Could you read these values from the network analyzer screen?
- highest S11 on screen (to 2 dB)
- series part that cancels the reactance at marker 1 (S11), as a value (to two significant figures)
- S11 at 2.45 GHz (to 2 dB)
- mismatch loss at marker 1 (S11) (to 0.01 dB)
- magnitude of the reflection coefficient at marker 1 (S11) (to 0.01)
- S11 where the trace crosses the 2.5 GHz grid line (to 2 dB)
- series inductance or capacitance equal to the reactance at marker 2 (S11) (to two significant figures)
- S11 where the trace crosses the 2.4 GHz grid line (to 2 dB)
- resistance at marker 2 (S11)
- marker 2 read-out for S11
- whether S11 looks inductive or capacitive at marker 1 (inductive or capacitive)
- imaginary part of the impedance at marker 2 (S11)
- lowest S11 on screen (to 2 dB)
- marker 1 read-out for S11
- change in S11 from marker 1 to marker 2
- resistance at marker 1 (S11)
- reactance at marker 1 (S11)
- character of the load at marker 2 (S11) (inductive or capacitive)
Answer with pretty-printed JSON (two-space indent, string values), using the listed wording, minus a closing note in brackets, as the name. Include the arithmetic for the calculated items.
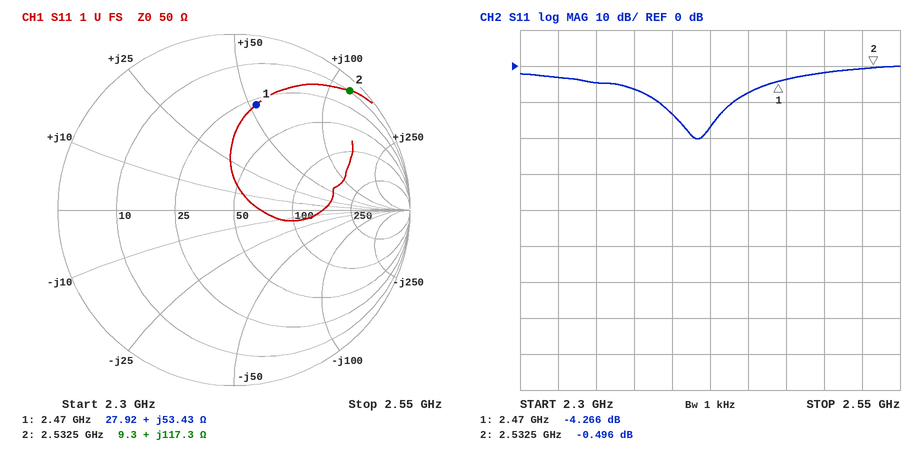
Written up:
{
  "highest S11 on screen": "0 dB",
  "series part that cancels the reactance at marker 1 (S11), as a value": "C = 1/(2π × 2.47 GHz × 53.43 Ω) ≈ 1.2 pF",
  "S11 at 2.45 GHz": "-8 dB",
  "mismatch loss at marker 1 (S11)": "−10 log10(1 − 10^(-4.266/10)) ≈ 2.04 dB",
  "magnitude of the reflection coefficient at marker 1 (S11)": "0.61",
  "S11 where the trace crosses the 2.5 GHz grid line": "-2 dB",
  "series inductance or capacitance equal to the reactance at marker 2 (S11)": "L = 117.3 Ω/(2π × 2.5325 GHz) ≈ 7.4 nH",
  "S11 where the trace crosses the 2.4 GHz grid line": "-14 dB",
  "resistance at marker 2": "9.3 Ω",
  "marker 2 read-out for S11": "-0.496 dB",
  "whether S11 looks inductive or capacitive at marker 1": "inductive",
  "imaginary part of the impedance at marker 2": "+117.3 Ω",
  "lowest S11 on screen": "-20 dB",
  "marker 1 read-out for S11": "-4.266 dB",
  "change in S11 from marker 1 to marker 2": "-0.496 − (-4.266) = 3.770 dB",
  "resistance at marker 1": "27.92 Ω",
  "reactance at marker 1": "+53.43 Ω",
  "character of the load at marker 2 (S11)": "inductive"
}
